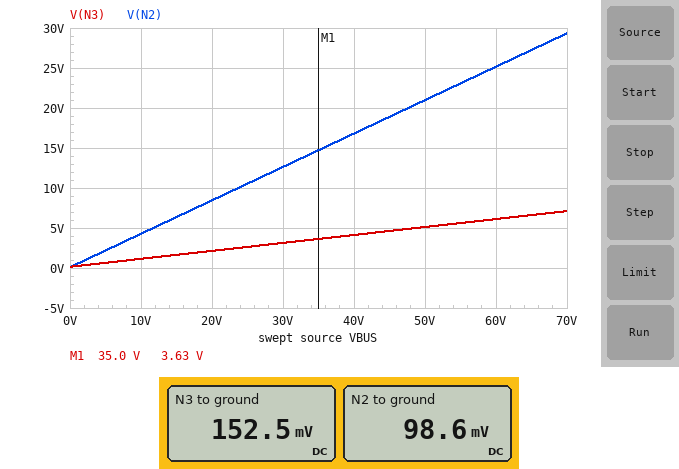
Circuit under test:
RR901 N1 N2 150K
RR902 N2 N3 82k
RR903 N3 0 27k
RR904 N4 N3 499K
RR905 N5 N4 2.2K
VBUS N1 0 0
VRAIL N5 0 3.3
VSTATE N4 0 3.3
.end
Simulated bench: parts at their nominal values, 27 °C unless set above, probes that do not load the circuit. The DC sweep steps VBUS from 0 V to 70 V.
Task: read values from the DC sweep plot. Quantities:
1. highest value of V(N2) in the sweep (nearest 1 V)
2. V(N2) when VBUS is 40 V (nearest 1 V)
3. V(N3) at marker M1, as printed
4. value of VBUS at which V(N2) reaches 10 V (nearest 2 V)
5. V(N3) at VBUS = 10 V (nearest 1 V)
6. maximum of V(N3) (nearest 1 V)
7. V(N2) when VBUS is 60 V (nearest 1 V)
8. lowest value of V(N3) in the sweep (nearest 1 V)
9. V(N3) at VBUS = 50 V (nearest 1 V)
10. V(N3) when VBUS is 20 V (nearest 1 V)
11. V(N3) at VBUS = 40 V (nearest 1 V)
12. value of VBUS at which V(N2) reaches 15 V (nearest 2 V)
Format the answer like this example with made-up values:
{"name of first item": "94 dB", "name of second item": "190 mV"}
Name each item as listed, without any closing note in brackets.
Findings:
{"highest value of V(N2) in the sweep": "29 V", "V(N2) when VBUS is 40 V": "17 V", "V(N3) at marker M1, as printed": "3.63 V", "value of VBUS at which V(N2) reaches 10 V": "24 V", "V(N3) at VBUS = 10 V": "1 V", "maximum of V(N3)": "7 V", "V(N2) when VBUS is 60 V": "25 V", "lowest value of V(N3) in the sweep": "0 V", "V(N3) at VBUS = 50 V": "5 V", "V(N3) when VBUS is 20 V": "2 V", "V(N3) at VBUS = 40 V": "4 V", "value of VBUS at which V(N2) reaches 15 V": "36 V"}
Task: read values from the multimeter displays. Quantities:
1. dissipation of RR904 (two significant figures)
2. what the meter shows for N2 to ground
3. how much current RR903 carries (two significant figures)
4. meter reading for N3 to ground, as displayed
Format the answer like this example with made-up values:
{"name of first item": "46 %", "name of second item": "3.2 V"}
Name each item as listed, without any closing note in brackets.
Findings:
{"dissipation of RR904": "20 µW", "what the meter shows for N2 to ground": "98.6 mV", "how much current RR903 carries": "5.6 µA", "meter reading for N3 to ground, as displayed": "152.5 mV"}
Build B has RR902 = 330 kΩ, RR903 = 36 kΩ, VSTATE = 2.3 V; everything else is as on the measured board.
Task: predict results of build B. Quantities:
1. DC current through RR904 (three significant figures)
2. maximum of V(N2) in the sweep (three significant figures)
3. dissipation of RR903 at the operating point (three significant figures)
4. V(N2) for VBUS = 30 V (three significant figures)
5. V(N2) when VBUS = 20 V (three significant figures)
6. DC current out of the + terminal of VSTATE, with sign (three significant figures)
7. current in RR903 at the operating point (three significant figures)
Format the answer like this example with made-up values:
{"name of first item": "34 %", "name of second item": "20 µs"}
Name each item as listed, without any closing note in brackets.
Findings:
{"DC current through RR904": "4.32 µA", "maximum of V(N2) in the sweep": "49.6 V", "dissipation of RR903 at the operating point": "581 nW", "V(N2) for VBUS = 30 V": "21.3 V", "V(N2) when VBUS = 20 V": "14.2 V", "DC current out of the + terminal of VSTATE, with sign": "-450 µA", "current in RR903 at the operating point": "4.02 µA"}
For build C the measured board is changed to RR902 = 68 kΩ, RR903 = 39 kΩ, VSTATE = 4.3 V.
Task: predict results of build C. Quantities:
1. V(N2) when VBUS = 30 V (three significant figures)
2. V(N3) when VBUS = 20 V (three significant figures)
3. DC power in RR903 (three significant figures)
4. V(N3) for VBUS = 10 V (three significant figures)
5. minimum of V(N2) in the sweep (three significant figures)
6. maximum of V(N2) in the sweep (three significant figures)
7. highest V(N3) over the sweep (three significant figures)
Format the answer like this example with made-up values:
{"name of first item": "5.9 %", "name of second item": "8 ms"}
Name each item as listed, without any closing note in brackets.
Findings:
{"V(N2) when VBUS = 30 V": "12.5 V", "V(N3) when VBUS = 20 V": "3.11 V", "DC power in RR903": "1.83 µW", "V(N3) for VBUS = 10 V": "1.69 V", "minimum of V(N2) in the sweep": "184 mV", "maximum of V(N2) in the sweep": "28.9 V", "highest V(N3) over the sweep": "10.2 V"}
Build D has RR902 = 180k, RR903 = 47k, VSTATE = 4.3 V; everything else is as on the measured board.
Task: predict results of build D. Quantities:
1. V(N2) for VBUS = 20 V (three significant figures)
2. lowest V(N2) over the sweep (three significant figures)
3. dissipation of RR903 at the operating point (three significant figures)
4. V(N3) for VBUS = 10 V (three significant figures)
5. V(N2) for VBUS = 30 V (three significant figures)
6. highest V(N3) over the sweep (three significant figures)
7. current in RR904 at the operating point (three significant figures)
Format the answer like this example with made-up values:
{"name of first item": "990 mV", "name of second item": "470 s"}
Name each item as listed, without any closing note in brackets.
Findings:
{"V(N2) for VBUS = 20 V": "12.1 V", "lowest V(N2) over the sweep": "149 mV", "dissipation of RR903 at the operating point": "2.28 µW", "V(N3) for VBUS = 10 V": "1.48 V", "V(N2) for VBUS = 30 V": "18.1 V", "highest V(N3) over the sweep": "8.39 V", "current in RR904 at the operating point": "7.96 µA"}
